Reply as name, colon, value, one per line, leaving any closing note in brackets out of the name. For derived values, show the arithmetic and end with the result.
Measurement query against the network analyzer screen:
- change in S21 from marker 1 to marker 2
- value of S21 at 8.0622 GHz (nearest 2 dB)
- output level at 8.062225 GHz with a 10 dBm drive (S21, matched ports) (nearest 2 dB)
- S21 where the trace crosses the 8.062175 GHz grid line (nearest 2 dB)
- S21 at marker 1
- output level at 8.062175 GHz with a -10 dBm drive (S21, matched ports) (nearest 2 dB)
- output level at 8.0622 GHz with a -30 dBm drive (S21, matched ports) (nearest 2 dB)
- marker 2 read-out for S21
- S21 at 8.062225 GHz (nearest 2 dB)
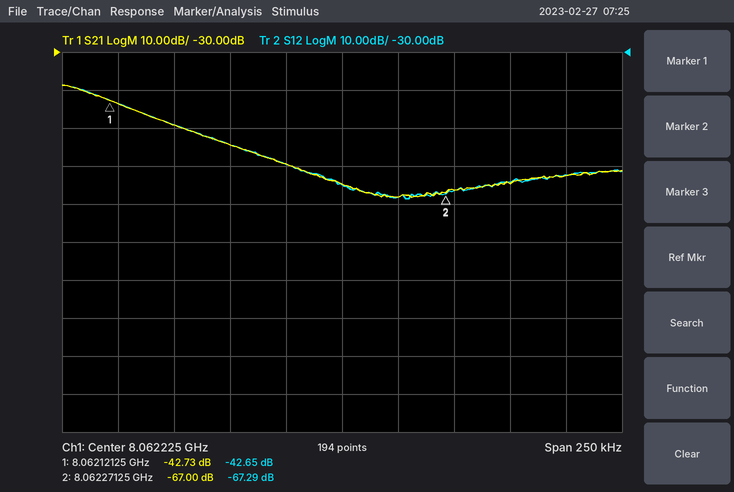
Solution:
change in S21 from marker 1 to marker 2: -67 − (-42.73) = -24.27 dB
value of S21 at 8.0622 GHz: -60 dB
output level at 8.062225 GHz with a 10 dBm drive (S21, matched ports): 10 dBm + (-64 dB) = -54 dBm
S21 where the trace crosses the 8.062175 GHz grid line: -54 dB
S21 at marker 1: -42.73 dB
output level at 8.062175 GHz with a -10 dBm drive (S21, matched ports): -10 dBm + (-54 dB) = -64 dBm
output level at 8.0622 GHz with a -30 dBm drive (S21, matched ports): -30 dBm + (-60 dB) = -90 dBm
marker 2 read-out for S21: -67.00 dB
S21 at 8.062225 GHz: -64 dB
